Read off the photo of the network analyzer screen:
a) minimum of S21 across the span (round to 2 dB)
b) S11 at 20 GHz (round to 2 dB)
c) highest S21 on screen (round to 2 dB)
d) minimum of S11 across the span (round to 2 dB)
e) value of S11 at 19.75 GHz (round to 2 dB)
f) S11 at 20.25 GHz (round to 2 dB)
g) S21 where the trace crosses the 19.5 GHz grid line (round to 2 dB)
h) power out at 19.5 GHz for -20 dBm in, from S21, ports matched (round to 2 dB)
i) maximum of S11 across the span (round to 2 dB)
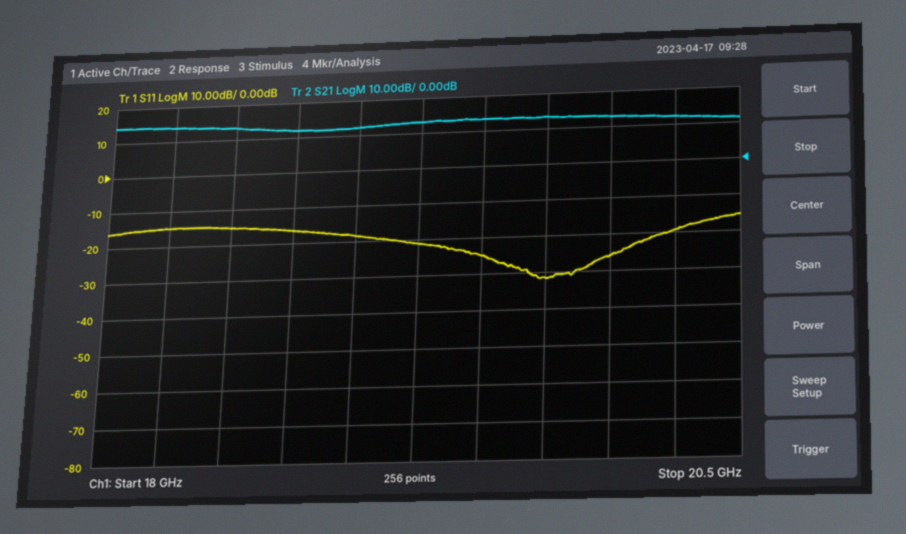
12 dB
-26 dB
14 dB
-32 dB
-32 dB
-20 dB
14 dB
-6 dBm
-14 dB
